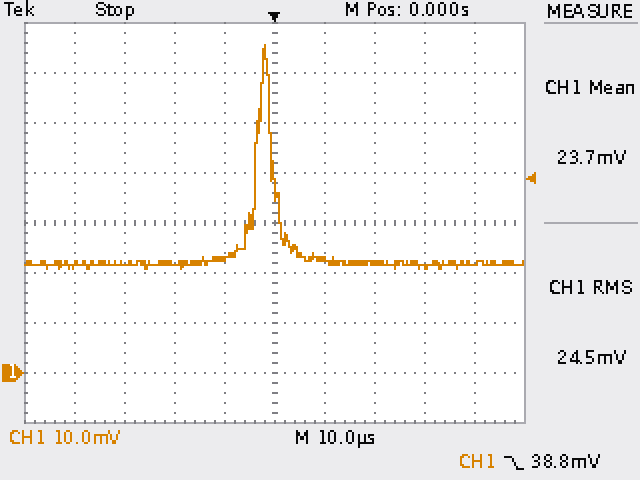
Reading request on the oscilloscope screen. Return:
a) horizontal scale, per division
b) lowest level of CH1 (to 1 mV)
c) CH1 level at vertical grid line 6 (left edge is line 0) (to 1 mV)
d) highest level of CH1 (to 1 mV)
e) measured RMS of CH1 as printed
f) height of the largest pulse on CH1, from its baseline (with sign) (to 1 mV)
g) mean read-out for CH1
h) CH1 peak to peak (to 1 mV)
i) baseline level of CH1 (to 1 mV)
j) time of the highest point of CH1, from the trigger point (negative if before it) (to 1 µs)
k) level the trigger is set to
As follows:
10 µs
21 mV
23 mV
66 mV
24.5 mV
+44 mV
23.7 mV
45 mV
22 mV
-2 µs
38.8 mV
